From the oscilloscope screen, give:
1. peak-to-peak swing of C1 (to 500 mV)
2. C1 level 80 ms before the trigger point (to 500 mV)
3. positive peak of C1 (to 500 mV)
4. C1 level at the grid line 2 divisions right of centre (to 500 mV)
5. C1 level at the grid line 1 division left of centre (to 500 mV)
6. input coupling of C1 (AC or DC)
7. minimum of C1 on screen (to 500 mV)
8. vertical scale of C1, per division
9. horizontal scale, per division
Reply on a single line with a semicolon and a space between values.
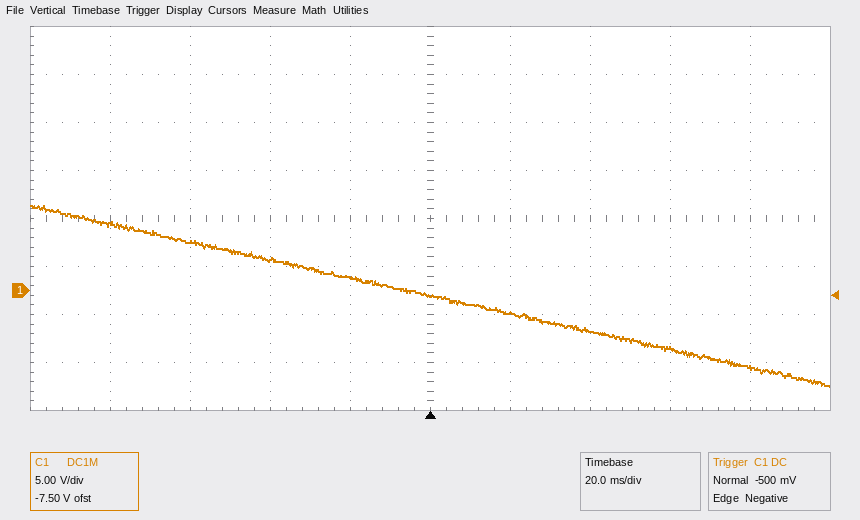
19.0 V; 7.0 V; 9.0 V; -4.0 V; 1.5 V; DC; -10.0 V; 5 V; 20 ms
